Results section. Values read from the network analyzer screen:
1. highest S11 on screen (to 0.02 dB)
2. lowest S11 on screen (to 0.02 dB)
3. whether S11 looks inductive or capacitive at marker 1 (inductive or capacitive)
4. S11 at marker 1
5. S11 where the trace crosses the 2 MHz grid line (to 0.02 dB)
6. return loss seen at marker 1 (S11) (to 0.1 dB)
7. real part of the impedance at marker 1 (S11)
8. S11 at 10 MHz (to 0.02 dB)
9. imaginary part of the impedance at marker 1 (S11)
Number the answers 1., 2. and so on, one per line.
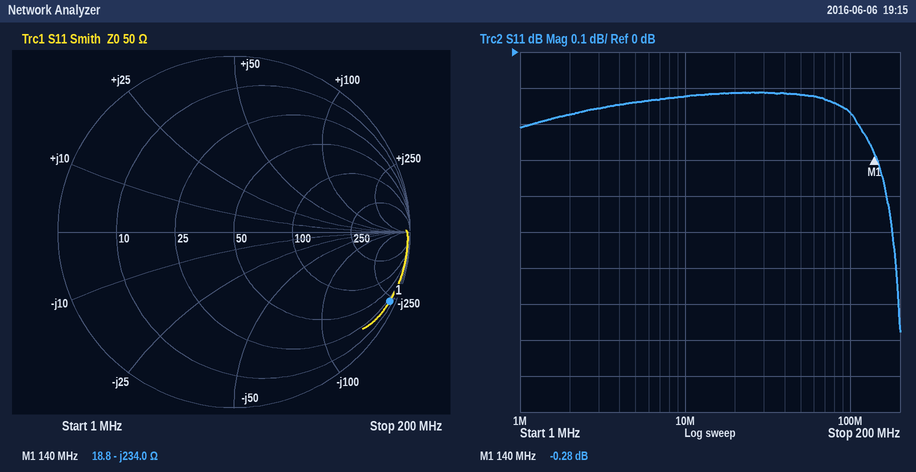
1. -0.12 dB
2. -0.78 dB
3. capacitive
4. -0.28 dB
5. -0.18 dB
6. 0.3 dB
7. 18.8 Ω
8. -0.12 dB
9. -234.0 Ω
